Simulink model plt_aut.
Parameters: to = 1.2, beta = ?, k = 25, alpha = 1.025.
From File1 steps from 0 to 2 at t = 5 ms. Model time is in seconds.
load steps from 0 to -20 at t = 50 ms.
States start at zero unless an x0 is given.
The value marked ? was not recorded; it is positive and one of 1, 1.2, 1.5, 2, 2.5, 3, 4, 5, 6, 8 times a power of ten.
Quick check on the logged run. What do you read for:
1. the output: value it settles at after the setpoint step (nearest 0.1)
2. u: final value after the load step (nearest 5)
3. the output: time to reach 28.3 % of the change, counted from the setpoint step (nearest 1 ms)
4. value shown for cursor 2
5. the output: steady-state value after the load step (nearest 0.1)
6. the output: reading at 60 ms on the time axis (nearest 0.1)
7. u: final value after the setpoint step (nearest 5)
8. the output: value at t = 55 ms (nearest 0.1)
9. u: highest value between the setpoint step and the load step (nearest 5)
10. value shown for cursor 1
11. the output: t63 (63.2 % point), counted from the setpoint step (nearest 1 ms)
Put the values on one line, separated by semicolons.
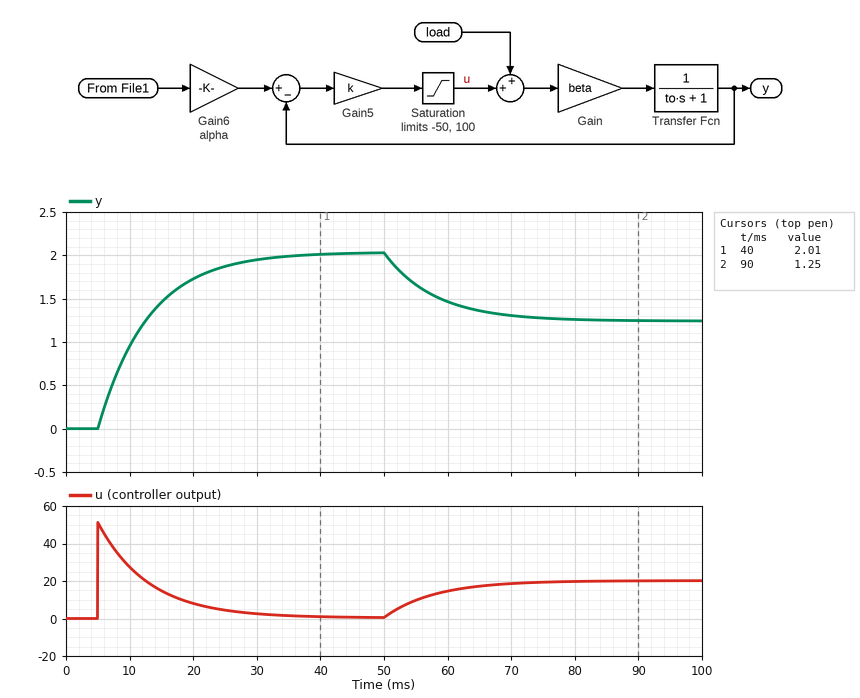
2.0; 20; 3 ms; 1.25; 1.2; 1.5; 0; 1.7; 50; 2.01; 8 ms
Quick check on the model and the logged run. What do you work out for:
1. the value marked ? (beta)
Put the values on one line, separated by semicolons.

6
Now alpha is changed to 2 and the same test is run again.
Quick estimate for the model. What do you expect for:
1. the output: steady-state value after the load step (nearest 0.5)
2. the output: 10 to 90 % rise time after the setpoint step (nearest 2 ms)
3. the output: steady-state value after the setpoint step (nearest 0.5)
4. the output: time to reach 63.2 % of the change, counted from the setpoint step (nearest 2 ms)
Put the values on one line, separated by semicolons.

3.0; 18 ms; 4.0; 8 ms
